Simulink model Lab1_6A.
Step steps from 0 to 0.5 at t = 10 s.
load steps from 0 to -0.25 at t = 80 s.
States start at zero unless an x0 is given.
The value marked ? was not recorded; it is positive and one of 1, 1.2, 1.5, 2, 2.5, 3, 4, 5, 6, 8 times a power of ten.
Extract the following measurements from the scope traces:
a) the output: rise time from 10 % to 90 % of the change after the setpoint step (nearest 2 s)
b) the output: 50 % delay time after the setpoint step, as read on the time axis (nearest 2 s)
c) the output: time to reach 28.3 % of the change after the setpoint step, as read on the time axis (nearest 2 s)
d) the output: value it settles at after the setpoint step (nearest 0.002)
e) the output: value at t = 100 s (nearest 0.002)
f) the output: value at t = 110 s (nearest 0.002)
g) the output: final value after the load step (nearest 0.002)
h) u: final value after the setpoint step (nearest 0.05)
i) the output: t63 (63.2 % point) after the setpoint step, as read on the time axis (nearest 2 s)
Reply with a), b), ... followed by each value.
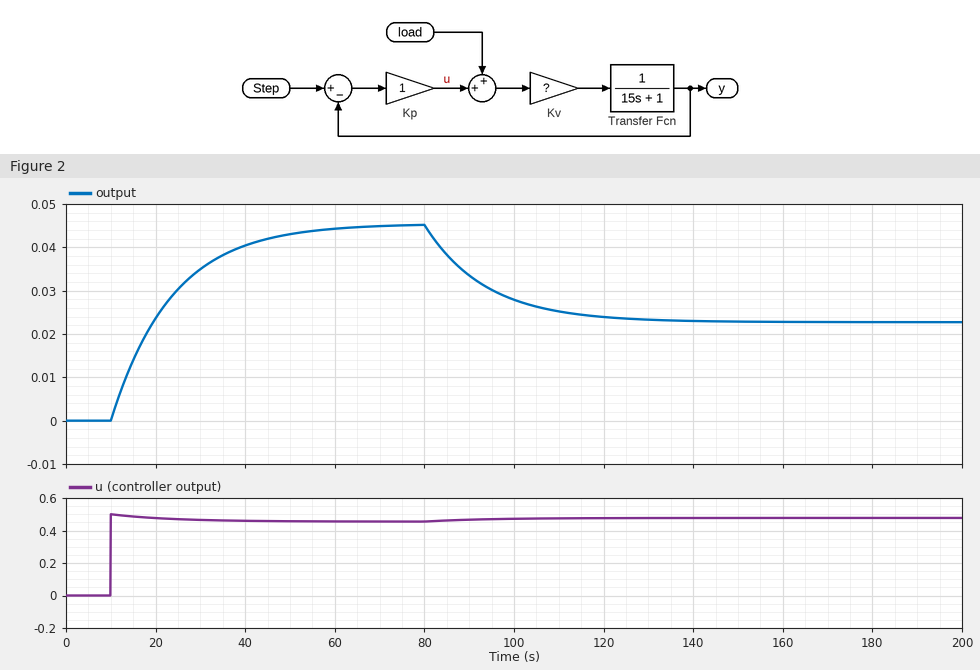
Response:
a) 30 s
b) 20 s
c) 14 s
d) 0.046
e) 0.028
f) 0.026
g) 0.022
h) 0.45
i) 24 s
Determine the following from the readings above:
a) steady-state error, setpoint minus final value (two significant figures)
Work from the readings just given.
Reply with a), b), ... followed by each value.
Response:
a) 0.45
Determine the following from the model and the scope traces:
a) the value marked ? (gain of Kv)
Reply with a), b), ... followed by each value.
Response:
a) 0.1
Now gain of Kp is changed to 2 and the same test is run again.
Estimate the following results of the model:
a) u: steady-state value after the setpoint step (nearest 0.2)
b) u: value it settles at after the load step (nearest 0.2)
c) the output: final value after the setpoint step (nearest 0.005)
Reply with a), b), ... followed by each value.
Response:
a) 0.8
b) 0.8
c) 0.085
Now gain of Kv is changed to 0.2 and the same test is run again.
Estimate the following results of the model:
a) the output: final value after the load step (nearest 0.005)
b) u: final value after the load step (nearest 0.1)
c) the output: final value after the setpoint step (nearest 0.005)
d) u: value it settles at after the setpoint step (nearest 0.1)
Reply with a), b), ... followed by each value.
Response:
a) 0.040
b) 0.5
c) 0.085
d) 0.4
